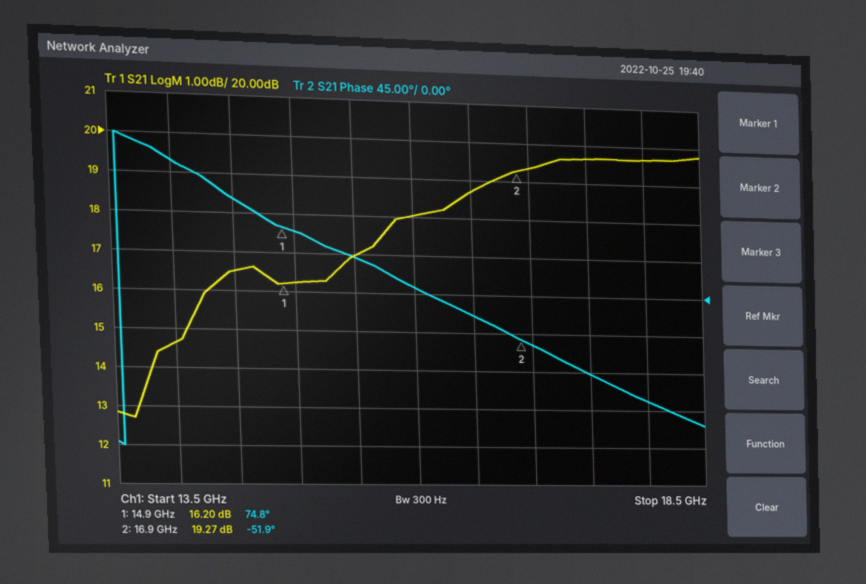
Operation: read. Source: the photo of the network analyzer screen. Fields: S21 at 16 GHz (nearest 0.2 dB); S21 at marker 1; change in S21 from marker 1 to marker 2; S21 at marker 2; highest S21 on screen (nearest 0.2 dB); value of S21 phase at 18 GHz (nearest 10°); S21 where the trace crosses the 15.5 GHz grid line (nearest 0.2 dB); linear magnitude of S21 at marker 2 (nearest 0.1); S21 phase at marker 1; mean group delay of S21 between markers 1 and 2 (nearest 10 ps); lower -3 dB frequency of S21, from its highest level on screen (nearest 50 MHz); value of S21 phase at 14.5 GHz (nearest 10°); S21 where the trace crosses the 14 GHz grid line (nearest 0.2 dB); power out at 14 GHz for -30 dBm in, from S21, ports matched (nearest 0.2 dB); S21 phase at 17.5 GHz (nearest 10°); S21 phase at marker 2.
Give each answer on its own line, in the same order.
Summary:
18.0 dB
16.20 dB
3.07 dB
19.27 dB
19.8 dB
-120°
17.0 dB
9.2
74.8°
180 ps
15.40 GHz
110°
14.6 dB
-15.4 dBm
-90°
-51.9°
